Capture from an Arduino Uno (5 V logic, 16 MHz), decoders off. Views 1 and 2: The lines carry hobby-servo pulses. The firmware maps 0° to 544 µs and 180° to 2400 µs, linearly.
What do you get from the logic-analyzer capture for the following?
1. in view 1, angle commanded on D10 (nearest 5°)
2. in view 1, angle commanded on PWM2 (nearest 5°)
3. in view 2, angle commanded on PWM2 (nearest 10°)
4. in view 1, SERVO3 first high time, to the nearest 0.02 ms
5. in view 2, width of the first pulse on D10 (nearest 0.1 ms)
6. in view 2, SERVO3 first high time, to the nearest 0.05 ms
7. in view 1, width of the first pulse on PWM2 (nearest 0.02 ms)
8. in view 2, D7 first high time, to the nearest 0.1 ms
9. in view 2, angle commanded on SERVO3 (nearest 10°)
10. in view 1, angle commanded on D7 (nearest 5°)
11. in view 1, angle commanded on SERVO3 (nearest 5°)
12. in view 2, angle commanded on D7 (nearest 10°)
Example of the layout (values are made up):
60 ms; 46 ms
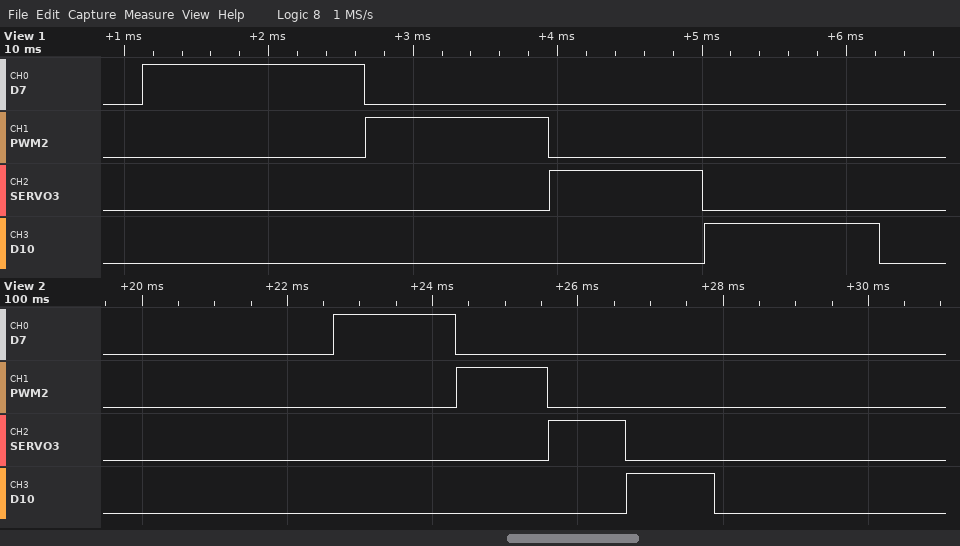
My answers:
65°; 70°; 70°; 1.06 ms; 1.2 ms; 1.05 ms; 1.26 ms; 1.7 ms; 50°; 95°; 50°; 110°
